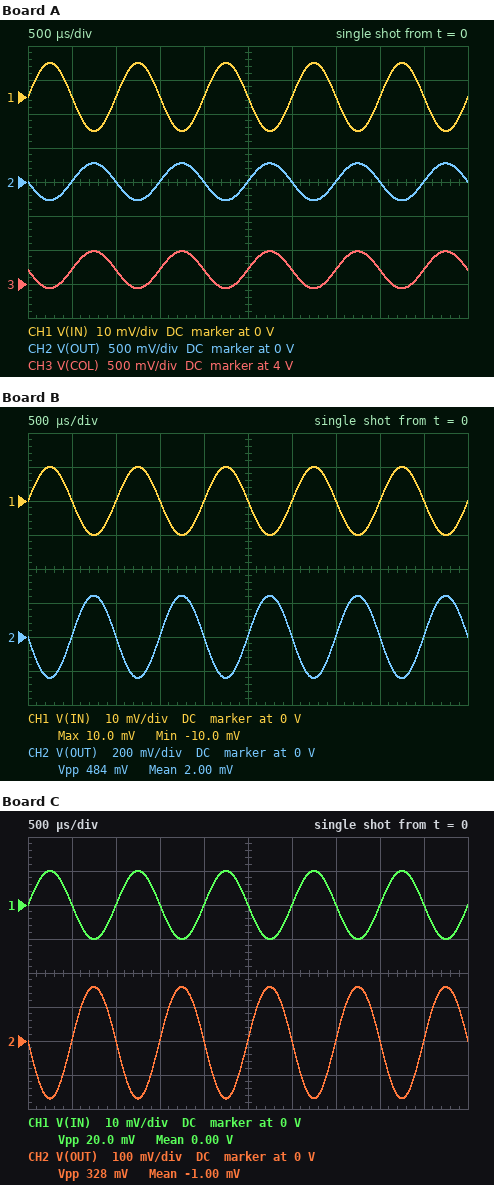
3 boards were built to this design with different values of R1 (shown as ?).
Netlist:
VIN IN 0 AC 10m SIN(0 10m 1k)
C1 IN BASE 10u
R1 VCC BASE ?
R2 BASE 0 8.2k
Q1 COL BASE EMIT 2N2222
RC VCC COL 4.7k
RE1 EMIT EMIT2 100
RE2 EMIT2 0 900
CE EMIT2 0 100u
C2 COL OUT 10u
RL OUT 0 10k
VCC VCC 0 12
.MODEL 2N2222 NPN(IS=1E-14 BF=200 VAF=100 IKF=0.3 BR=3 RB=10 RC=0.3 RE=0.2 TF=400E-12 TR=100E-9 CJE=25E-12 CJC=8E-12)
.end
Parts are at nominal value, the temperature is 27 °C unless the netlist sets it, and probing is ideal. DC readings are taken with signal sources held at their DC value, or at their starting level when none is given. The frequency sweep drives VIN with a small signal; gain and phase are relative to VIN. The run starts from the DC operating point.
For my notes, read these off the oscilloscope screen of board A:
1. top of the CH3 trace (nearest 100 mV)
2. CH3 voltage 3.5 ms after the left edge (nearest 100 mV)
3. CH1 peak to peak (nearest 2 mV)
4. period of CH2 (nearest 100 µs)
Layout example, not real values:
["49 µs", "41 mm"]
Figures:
["4.5 V", "4.2 V", "20 mV", "1.0 ms"]
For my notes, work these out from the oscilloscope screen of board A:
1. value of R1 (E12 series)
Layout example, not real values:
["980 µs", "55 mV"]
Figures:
["33 kΩ"]
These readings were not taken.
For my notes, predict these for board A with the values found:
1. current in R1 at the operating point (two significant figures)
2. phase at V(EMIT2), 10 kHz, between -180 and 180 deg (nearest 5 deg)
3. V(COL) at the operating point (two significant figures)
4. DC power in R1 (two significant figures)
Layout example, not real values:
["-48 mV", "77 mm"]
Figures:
["290 µA", "-90 deg", "4.2 V", "2.8 mW"]
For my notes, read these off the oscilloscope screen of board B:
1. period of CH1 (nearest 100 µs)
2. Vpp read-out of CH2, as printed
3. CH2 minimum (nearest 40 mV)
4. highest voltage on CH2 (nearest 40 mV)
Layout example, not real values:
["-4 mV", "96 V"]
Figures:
["1.0 ms", "484 mV", "-240 mV", "240 mV"]
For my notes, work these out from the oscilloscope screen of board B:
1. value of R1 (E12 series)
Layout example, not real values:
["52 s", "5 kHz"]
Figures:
["56 kΩ"]
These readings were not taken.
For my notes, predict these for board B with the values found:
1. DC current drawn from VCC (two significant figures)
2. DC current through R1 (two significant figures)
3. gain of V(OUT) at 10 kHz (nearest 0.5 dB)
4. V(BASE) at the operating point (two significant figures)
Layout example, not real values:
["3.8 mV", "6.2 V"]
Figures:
["1.0 mA", "190 µA", "27.5 dB", "1.5 V"]
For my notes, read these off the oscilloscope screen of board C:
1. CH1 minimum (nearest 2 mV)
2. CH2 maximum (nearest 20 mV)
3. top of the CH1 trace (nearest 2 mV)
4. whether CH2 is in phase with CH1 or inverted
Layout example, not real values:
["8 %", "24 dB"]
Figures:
["-10 mV", "160 mV", "10 mV", "inverted"]
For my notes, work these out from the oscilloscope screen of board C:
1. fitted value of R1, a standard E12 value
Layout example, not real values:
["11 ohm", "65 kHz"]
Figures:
["100 kΩ"]
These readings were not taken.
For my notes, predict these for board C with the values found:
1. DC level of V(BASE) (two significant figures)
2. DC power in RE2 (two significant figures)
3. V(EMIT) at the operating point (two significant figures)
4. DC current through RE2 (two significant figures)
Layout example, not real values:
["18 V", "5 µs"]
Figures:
["900 mV", "71 µW", "280 mV", "280 µA"]
